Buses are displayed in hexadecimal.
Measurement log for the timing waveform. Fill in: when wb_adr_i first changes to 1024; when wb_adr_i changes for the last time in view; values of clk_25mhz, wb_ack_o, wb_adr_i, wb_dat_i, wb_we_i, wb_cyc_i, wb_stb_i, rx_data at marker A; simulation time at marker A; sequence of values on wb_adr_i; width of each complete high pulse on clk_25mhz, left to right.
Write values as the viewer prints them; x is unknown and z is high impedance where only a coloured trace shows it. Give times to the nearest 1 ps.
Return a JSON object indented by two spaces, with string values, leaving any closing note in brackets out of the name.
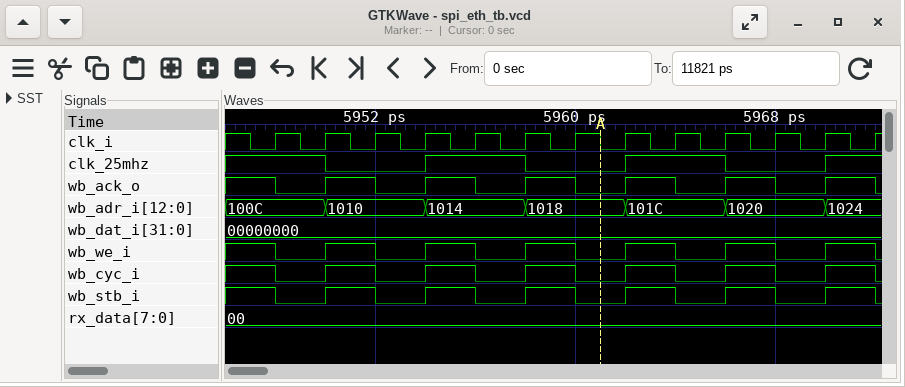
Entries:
{
  "when wb_adr_i first changes to 1024": "5970 ps",
  "when wb_adr_i changes for the last time in view": "5970 ps",
  "values of clk_25mhz, wb_ack_o, wb_adr_i, wb_dat_i, wb_we_i, wb_cyc_i, wb_stb_i, rx_data at marker A": "clk_25mhz=0, wb_ack_o=0, wb_adr_i=1018, wb_dat_i=00000000, wb_we_i=0, wb_cyc_i=0, wb_stb_i=0, rx_data=00",
  "simulation time at marker A": "5961 ps",
  "sequence of values on wb_adr_i": "100C, 1010, 1014, 1018, 101C, 1020, 1024",
  "width of each complete high pulse on clk_25mhz, left to right": "4 ps, 4 ps"
}
